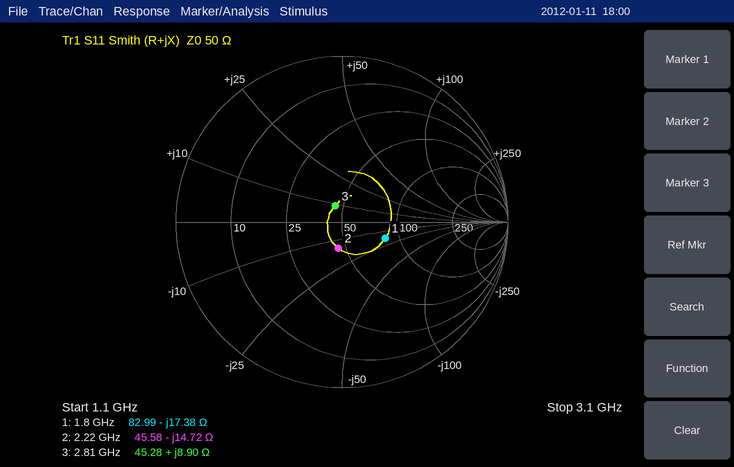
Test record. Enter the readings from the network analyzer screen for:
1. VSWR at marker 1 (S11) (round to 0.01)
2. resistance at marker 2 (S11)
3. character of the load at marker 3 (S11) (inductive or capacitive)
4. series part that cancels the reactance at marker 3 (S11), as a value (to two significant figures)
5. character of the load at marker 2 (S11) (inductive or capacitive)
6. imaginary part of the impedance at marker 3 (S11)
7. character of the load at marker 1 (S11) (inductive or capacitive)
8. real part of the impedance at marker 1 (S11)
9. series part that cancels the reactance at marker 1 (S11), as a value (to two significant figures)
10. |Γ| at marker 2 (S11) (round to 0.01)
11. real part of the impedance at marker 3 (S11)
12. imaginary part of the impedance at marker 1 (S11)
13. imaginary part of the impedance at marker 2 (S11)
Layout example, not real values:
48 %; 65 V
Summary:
1.77; 45.58 Ω; inductive; 6.4 pF; capacitive; +8.90 Ω; capacitive; 82.99 Ω; 1.5 nH; 0.16; 45.28 Ω; -17.38 Ω; -14.72 Ω
